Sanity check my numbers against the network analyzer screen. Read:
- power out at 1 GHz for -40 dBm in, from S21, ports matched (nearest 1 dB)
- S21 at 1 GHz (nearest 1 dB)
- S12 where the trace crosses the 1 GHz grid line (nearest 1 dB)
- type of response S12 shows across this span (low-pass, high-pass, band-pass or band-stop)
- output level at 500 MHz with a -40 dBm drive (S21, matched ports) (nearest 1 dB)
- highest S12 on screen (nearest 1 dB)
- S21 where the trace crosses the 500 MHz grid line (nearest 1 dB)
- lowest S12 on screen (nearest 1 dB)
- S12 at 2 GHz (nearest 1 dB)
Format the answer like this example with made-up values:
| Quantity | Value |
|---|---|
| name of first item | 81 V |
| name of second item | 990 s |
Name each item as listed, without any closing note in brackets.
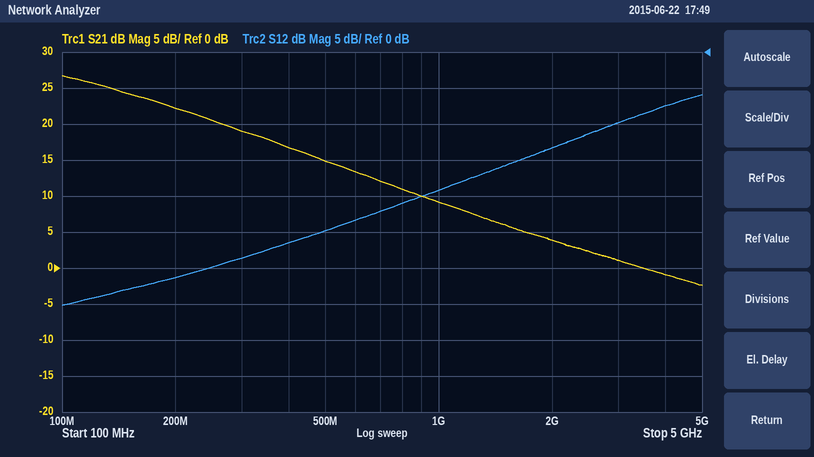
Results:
| Quantity | Value |
|---|---|
| power out at 1 GHz for -40 dBm in, from S21, ports matched | -31 dBm |
| S21 at 1 GHz | 9 dB |
| S12 where the trace crosses the 1 GHz grid line | -19 dB |
| type of response S12 shows across this span | high-pass |
| output level at 500 MHz with a -40 dBm drive (S21, matched ports) | -25 dBm |
| highest S12 on screen | -6 dB |
| S21 where the trace crosses the 500 MHz grid line | 15 dB |
| lowest S12 on screen | -35 dB |
| S12 at 2 GHz | -13 dB |
